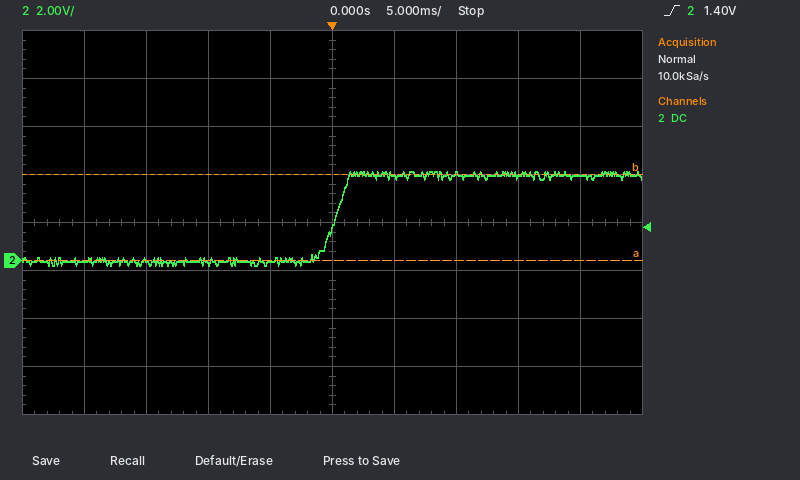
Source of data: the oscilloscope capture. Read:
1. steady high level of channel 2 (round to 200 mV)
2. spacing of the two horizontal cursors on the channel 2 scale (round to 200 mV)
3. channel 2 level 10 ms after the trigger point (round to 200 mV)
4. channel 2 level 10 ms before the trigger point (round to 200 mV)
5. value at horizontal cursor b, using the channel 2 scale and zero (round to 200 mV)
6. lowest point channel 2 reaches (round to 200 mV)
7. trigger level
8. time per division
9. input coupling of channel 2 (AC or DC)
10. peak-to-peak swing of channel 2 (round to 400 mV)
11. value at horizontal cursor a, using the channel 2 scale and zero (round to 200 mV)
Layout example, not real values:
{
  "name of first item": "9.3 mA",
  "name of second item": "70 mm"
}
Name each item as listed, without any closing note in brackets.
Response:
{
  "steady high level of channel 2": "3.6 V",
  "spacing of the two horizontal cursors on the channel 2 scale": "3.6 V",
  "channel 2 level 10 ms after the trigger point": "3.6 V",
  "channel 2 level 10 ms before the trigger point": "0.0 V",
  "value at horizontal cursor b, using the channel 2 scale and zero": "3.6 V",
  "lowest point channel 2 reaches": "-200 mV",
  "trigger level": "1.40 V",
  "time per division": "5 ms",
  "input coupling of channel 2": "DC",
  "peak-to-peak swing of channel 2": "4.0 V",
  "value at horizontal cursor a, using the channel 2 scale and zero": "0.0 V"
}
